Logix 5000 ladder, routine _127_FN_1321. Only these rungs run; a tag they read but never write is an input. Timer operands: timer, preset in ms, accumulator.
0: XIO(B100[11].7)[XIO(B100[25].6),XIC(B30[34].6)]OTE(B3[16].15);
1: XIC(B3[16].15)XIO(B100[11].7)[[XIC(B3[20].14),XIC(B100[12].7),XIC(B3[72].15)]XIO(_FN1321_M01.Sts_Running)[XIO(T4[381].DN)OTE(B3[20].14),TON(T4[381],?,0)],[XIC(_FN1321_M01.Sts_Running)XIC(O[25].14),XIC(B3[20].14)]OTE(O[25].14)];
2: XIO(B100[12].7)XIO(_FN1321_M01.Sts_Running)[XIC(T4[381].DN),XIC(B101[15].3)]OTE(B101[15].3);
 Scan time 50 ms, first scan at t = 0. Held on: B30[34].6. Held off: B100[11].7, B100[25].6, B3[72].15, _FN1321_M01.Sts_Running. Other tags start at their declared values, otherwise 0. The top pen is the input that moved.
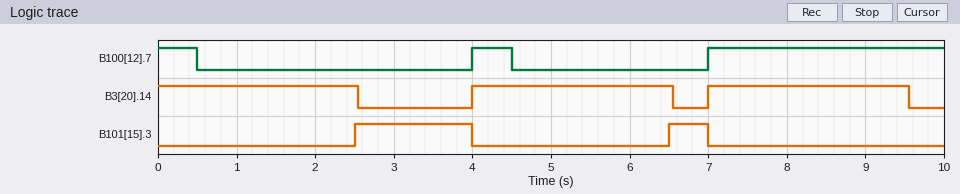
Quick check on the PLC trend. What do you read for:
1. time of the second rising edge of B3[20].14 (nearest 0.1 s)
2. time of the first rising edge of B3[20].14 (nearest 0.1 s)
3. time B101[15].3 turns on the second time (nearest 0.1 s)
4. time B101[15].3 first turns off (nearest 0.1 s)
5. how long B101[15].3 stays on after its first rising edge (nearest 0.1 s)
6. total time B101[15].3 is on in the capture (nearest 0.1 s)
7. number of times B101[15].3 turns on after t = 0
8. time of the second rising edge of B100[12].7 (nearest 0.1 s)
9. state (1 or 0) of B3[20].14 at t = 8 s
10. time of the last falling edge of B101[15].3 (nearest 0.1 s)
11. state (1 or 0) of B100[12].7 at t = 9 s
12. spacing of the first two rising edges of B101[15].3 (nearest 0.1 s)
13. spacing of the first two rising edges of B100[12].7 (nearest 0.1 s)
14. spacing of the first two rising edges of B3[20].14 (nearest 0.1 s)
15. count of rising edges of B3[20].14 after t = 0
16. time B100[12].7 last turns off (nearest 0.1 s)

7.0 s
4.0 s
6.5 s
4.0 s
1.5 s
2.0 s
2
7.0 s
1
7.0 s
1
4.0 s
3.0 s
3.0 s
2
4.5 s
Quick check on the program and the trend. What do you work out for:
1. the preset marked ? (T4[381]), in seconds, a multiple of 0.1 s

2.5 s
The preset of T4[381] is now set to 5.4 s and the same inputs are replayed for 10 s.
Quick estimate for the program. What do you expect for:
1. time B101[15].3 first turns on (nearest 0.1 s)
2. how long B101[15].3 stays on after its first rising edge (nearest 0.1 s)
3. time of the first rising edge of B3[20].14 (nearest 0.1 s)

5.4 s
1.6 s
7.0 s
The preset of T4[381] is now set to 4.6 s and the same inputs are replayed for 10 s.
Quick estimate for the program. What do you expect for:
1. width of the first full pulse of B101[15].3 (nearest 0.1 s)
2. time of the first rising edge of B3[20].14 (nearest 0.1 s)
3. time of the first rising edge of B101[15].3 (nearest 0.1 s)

2.4 s
7.0 s
4.6 s
